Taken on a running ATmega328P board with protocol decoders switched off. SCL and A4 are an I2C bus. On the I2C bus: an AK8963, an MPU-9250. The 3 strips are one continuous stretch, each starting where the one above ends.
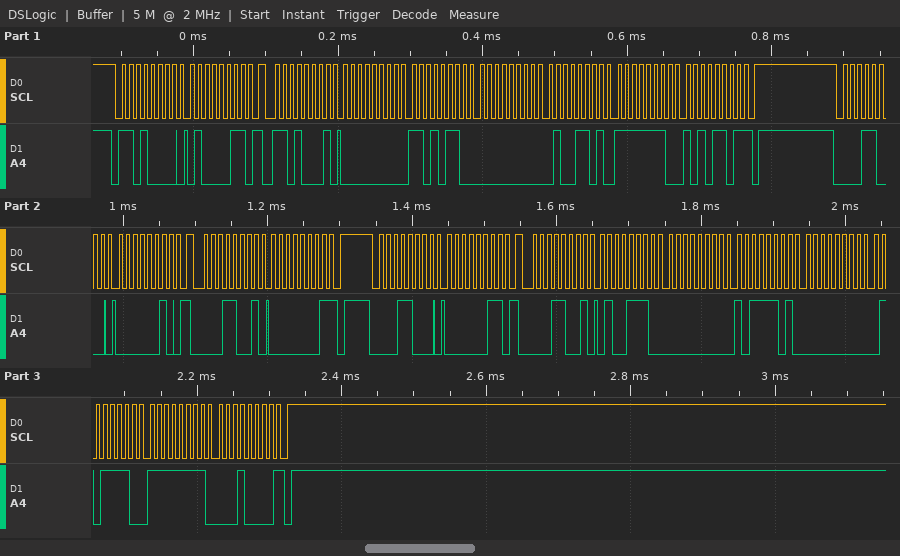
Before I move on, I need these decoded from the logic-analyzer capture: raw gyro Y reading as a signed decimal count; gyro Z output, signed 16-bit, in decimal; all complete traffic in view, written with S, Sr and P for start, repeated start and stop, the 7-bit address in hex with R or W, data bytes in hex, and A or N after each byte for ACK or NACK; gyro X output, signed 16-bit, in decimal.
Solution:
77
-339
S 68W A 43 A Sr 68R A 00 A D6 A 00 A 4D A FE A AD N P S 0CW A 02 A Sr 0CR A 01 N P S 0CW A 03 A Sr 0CR A 4E A 00 A BD A 00 A 5E A FF A 10 N P
214
